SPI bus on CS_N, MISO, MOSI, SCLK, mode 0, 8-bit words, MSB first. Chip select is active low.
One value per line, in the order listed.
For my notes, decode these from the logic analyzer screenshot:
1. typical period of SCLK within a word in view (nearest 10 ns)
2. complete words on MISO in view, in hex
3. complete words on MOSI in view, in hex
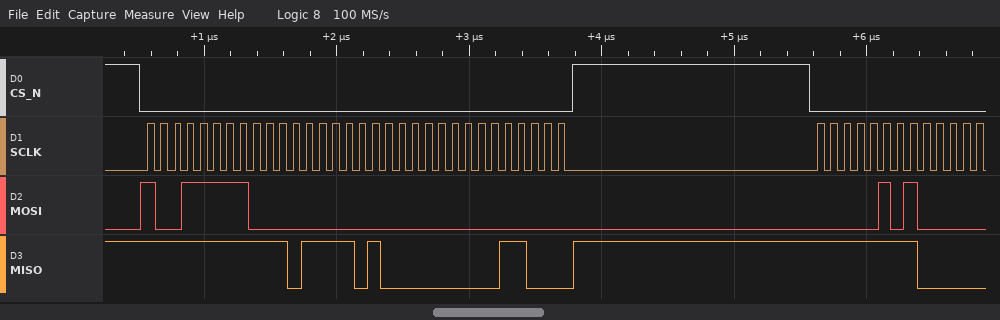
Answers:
100 ns
FF, EF, 40, 18, FF
9F, 00, 00, 00, 05
